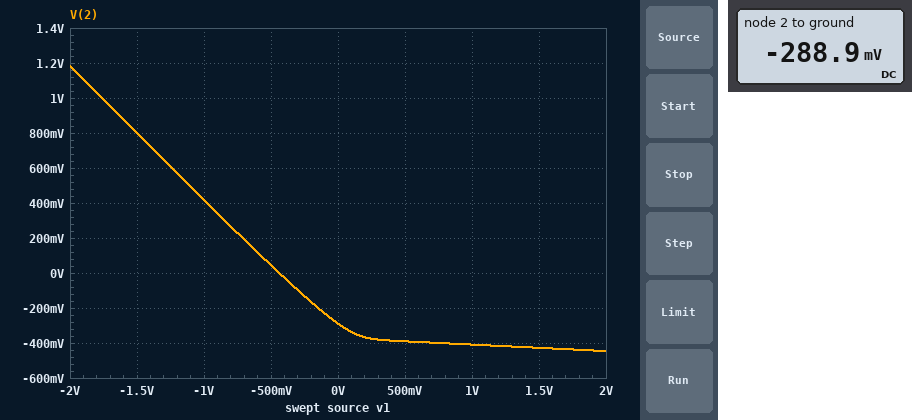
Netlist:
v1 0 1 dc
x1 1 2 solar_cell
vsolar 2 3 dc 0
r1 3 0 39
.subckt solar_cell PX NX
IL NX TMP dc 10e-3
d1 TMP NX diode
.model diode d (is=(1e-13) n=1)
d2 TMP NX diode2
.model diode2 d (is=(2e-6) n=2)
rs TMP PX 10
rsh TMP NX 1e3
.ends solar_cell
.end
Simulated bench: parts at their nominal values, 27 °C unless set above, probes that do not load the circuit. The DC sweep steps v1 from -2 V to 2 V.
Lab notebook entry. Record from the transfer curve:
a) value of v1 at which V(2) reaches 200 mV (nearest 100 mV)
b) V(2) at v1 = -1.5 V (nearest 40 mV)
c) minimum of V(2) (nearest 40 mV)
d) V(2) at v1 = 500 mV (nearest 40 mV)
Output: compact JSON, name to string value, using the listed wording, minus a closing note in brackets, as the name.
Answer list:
{"value of v1 at which V(2) reaches 200 mV": "-700 mV", "V(2) at v1 = -1.5 V": "800 mV", "minimum of V(2)": "-440 mV", "V(2) at v1 = 500 mV": "-400 mV"}
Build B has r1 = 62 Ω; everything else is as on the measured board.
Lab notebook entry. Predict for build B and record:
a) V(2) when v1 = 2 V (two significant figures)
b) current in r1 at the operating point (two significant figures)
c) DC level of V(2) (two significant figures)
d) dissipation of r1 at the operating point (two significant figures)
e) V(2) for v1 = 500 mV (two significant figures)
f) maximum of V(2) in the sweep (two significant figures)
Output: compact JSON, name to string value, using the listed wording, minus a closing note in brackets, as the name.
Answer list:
{"V(2) when v1 = 2 V": "-690 mV", "current in r1 at the operating point": "5.5 mA", "DC level of V(2)": "-340 mV", "dissipation of r1 at the operating point": "1.9 mW", "V(2) for v1 = 500 mV": "-600 mV", "maximum of V(2) in the sweep": "1.3 V"}
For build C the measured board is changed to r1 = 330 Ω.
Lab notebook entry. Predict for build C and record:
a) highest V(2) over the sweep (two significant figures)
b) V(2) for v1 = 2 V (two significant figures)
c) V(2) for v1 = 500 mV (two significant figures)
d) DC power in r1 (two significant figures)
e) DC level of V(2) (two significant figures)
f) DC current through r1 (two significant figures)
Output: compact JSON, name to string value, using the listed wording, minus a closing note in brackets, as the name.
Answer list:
{"highest V(2) over the sweep": "1.5 V", "V(2) for v1 = 2 V": "-2.3 V", "V(2) for v1 = 500 mV": "-890 mV", "DC power in r1": "530 µW", "DC level of V(2)": "-420 mV", "DC current through r1": "1.3 mA"}
